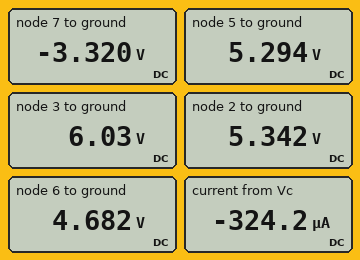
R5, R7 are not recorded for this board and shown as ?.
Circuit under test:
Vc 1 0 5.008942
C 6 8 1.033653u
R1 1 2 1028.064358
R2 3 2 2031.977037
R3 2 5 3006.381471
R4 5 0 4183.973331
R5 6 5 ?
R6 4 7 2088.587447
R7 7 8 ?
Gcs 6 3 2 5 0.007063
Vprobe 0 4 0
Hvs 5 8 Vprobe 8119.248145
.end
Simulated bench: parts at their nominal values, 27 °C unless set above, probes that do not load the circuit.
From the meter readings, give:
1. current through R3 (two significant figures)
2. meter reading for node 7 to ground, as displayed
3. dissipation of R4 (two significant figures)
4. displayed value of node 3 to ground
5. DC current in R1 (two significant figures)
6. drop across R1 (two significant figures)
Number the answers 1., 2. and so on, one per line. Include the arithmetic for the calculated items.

1. (5.342 V - 5.294 V) / 3.006 kΩ = 16 µA
2. -3.320 V
3. (5.294 V)^2 / 4.184 kΩ = 6.7 mW
4. 6.03 V
5. (5.342 V - 5.009 V) / 1.028 kΩ = 320 µA
6. 5.342 V - 5.009 V = 330 mV
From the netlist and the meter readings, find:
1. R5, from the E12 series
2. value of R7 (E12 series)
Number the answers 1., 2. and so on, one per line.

1. 1.8 kΩ
2. 2.7 kΩ
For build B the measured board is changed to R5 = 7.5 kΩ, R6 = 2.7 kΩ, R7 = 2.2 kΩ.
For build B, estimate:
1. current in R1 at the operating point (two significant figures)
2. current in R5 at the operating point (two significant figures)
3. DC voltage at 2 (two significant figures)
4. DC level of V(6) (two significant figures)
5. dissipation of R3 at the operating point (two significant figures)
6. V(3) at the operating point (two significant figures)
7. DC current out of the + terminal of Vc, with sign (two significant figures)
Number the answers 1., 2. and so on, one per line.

1. 380 µA
2. 400 µA
3. 5.4 V
4. 2.3 V
5. 1.1 µW
6. 6.2 V
7. -380 µA
